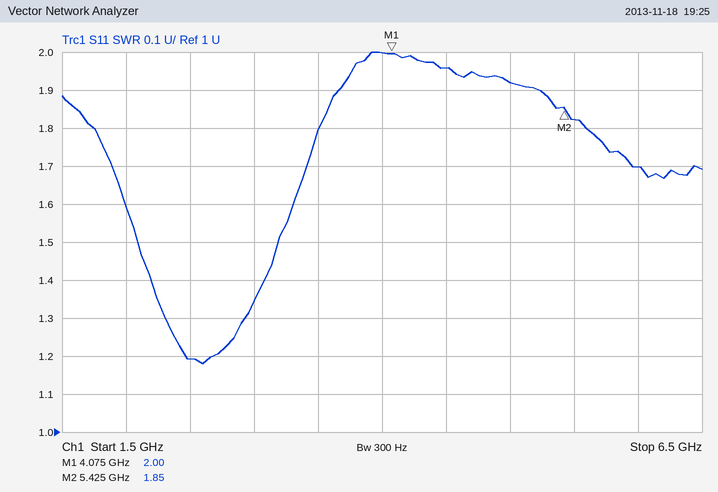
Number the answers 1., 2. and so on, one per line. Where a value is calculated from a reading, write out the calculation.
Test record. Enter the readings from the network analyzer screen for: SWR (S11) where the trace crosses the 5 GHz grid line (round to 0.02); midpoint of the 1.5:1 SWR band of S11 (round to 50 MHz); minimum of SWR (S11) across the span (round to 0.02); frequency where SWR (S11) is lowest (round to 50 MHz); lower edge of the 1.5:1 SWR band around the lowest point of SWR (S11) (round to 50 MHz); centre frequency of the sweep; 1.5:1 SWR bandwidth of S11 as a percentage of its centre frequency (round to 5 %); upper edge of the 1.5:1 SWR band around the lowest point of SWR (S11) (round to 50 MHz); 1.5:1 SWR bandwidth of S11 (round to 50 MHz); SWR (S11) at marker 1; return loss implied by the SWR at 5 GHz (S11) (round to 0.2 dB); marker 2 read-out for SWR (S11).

1. 1.92
2. 2.65 GHz
3. 1.18
4. 2.60 GHz
5. 2.10 GHz
6. 4 GHz
7. 1.1 GHz / 2.65 GHz ≈ 41.5 %, so 40 % to the nearest 5 %
8. 3.20 GHz
9. 3.20 GHz − 2.10 GHz = 1.10 GHz
10. 2.00
11. −20 log10((1.92 − 1)/(1.92 + 1)) ≈ 10.0 dB
12. 1.85
